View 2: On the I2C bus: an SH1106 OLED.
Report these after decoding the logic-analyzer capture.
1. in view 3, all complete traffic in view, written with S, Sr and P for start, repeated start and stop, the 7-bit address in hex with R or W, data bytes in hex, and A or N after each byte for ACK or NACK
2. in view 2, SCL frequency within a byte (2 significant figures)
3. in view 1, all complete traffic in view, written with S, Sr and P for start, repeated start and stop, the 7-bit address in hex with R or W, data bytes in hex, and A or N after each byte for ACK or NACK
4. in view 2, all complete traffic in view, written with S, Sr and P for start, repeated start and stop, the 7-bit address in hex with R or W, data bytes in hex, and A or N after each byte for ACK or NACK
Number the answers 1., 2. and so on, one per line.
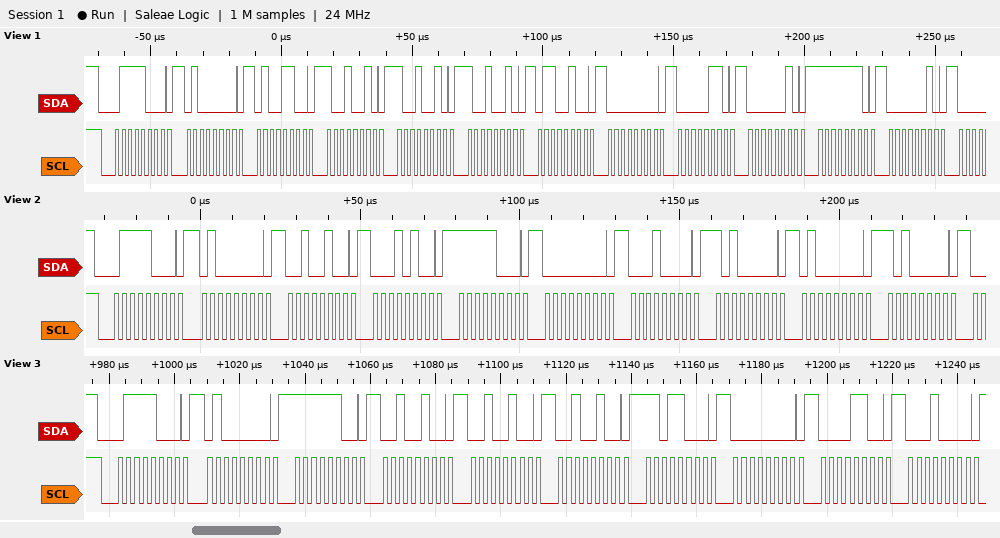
1. S 3CW A 40 A FC A 24 A 24 A 24 A D8 A 00 A 0C A 10 A
2. 400 kHz
3. S 3CW A 40 A 4C A 92 A 92 A 92 A 64 A 00 A 06 A 02 A FE A 02 A
4. S 3CW A 40 A 24 A 14 A F8 A 00 A 10 A A0 A 40 A A0 A
